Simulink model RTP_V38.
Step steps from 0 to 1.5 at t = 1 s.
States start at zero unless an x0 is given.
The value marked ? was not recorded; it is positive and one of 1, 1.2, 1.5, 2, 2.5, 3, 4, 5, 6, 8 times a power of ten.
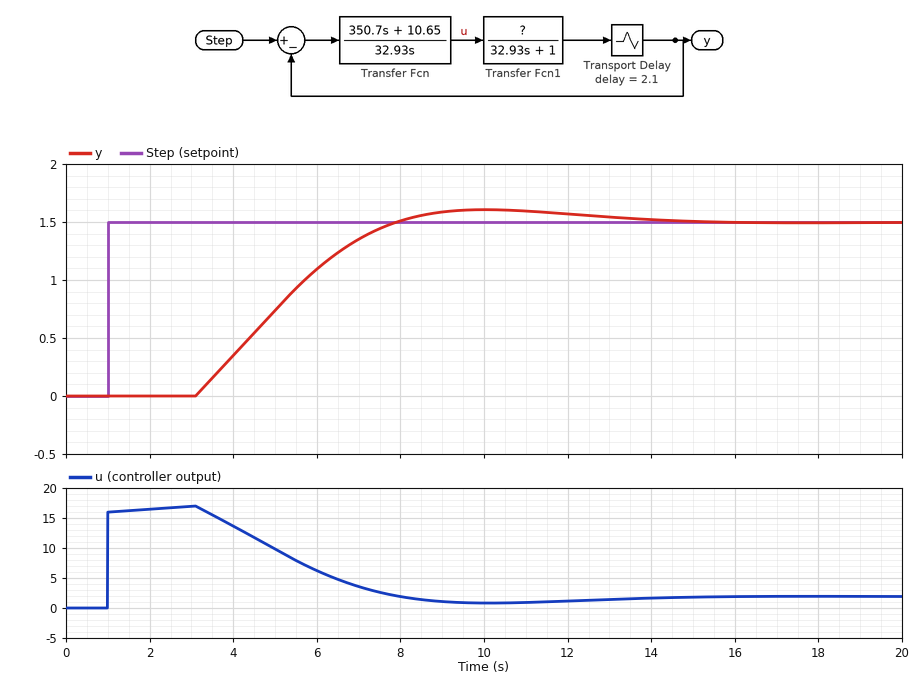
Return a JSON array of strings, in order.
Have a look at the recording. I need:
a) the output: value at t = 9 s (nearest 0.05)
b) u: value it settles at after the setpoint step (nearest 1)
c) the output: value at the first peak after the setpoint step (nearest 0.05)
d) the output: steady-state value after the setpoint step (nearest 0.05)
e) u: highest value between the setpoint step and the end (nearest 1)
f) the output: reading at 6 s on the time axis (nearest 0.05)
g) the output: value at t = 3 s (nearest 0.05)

["1.60", "2", "1.60", "1.50", "17", "1.10", "0.00"]
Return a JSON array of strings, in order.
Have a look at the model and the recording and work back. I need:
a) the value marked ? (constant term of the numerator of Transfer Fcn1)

["0.8"]
